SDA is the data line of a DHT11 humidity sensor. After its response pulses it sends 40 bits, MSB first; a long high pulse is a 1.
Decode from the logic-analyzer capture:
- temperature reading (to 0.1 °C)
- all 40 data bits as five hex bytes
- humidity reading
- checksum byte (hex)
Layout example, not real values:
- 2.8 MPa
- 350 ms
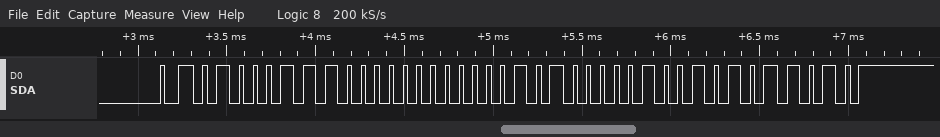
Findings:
- 10.9 °C
- 47 00 0A 09 5A
- 71 %
- 0x5A
